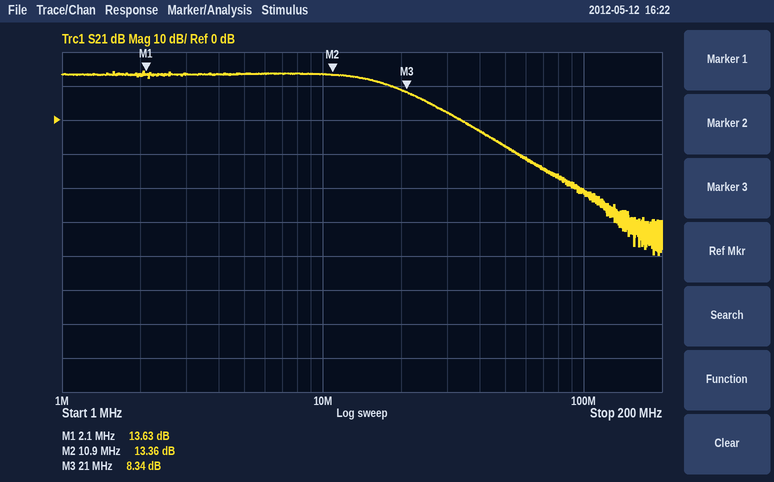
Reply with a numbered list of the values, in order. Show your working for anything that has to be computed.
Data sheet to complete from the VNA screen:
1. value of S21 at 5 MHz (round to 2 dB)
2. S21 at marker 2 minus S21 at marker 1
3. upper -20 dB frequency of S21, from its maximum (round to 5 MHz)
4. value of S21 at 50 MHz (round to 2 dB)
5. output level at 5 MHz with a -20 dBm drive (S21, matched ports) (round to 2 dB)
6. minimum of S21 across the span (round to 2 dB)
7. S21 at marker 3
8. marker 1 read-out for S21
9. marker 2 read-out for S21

1. 14 dB
2. 13.36 − (13.63) = -0.27 dB
3. 45 MHz
4. -8 dB
5. -20 dBm + (14 dB) = -6 dBm
6. -40 dB
7. 8.34 dB
8. 13.63 dB
9. 13.36 dB
